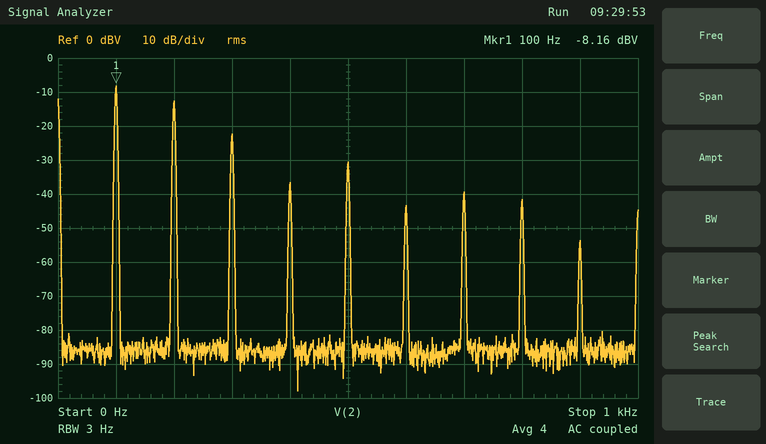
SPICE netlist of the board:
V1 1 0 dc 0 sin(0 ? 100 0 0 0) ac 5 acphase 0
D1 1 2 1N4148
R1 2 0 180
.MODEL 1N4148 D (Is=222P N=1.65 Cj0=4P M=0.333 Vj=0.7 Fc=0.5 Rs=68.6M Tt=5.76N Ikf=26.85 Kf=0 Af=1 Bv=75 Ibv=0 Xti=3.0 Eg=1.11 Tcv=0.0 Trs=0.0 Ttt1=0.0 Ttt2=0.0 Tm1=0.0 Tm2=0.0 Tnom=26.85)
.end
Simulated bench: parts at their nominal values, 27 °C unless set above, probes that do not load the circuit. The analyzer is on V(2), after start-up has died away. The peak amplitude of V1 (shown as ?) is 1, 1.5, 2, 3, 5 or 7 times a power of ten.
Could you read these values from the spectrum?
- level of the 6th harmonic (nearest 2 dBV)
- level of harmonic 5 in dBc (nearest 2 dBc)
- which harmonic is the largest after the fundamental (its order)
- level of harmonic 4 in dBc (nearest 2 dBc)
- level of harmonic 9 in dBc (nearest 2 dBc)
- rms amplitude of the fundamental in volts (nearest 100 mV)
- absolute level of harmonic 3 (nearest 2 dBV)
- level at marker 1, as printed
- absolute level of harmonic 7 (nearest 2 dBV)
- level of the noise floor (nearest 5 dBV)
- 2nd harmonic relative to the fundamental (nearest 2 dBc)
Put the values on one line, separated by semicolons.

-44 dBV; -22 dBc; 2; -28 dBc; -46 dBc; 400 mV; -22 dBV; -8.16 dBV; -40 dBV; -85 dBV; -4 dBc
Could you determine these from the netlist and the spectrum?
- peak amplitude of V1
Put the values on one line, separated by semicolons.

2 V
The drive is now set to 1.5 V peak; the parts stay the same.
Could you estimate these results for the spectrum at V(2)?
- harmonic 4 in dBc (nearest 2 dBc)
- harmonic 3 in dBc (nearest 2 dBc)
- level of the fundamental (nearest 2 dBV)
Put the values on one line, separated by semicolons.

-36 dBc; -12 dBc; -12 dBV
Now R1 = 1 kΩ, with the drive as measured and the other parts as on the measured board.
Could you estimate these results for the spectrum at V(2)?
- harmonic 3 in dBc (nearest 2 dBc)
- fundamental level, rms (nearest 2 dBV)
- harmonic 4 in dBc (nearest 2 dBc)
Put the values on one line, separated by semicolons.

-16 dBc; -8 dBV; -26 dBc
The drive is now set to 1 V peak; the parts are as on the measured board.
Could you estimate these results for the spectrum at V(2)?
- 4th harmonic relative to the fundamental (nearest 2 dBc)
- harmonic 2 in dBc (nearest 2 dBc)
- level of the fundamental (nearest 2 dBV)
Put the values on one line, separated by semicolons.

-16 dBc; -2 dBc; -22 dBV
